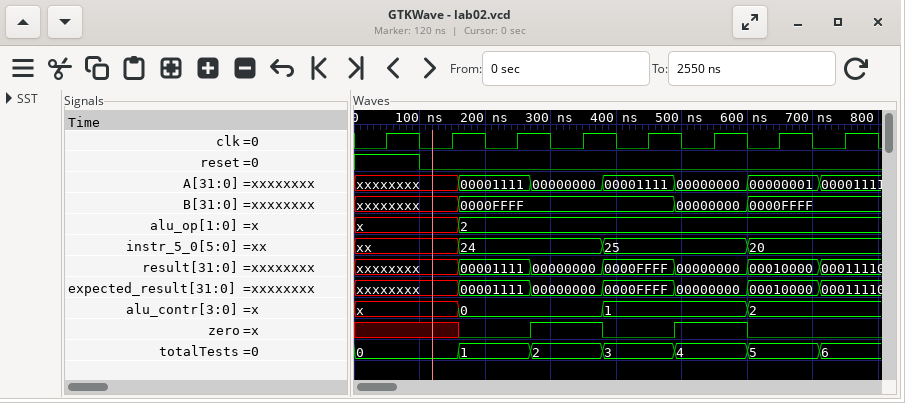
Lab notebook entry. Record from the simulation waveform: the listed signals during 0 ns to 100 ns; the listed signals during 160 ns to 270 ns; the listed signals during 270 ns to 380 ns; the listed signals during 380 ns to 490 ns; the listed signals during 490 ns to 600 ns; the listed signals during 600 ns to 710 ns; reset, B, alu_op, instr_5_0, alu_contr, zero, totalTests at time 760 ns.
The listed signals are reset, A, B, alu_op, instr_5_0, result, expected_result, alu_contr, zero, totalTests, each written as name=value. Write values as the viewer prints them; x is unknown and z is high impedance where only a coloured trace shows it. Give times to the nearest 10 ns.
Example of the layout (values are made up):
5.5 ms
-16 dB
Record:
reset=1, A=xxxxxxxx, B=xxxxxxxx, alu_op=x, instr_5_0=xx, result=xxxxxxxx, expected_result=xxxxxxxx, alu_contr=x, zero=x, totalTests=0
reset=0, A=00001111, B=0000FFFF, alu_op=2, instr_5_0=24, result=00001111, expected_result=00001111, alu_contr=0, zero=0, totalTests=1
reset=0, A=00000000, B=0000FFFF, alu_op=2, instr_5_0=24, result=00000000, expected_result=00000000, alu_contr=0, zero=1, totalTests=2
reset=0, A=00001111, B=0000FFFF, alu_op=2, instr_5_0=25, result=0000FFFF, expected_result=0000FFFF, alu_contr=1, zero=0, totalTests=3
reset=0, A=00000000, B=00000000, alu_op=2, instr_5_0=25, result=00000000, expected_result=00000000, alu_contr=1, zero=1, totalTests=4
reset=0, A=00000001, B=0000FFFF, alu_op=2, instr_5_0=20, result=00010000, expected_result=00010000, alu_contr=2, zero=0, totalTests=5
reset=0, B=0000FFFF, alu_op=2, instr_5_0=20, alu_contr=2, zero=0, totalTests=6
